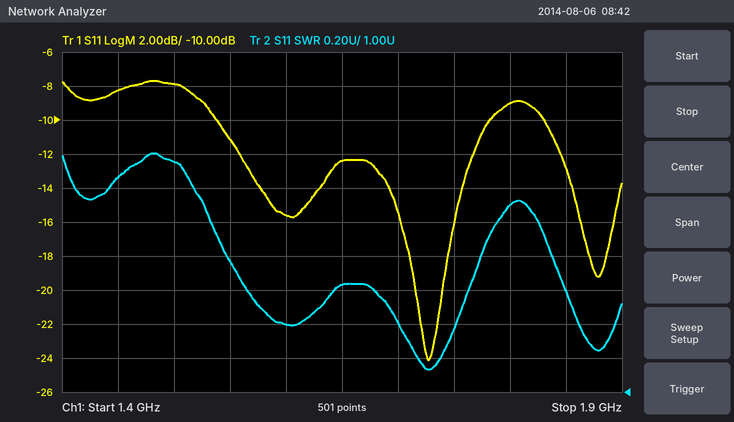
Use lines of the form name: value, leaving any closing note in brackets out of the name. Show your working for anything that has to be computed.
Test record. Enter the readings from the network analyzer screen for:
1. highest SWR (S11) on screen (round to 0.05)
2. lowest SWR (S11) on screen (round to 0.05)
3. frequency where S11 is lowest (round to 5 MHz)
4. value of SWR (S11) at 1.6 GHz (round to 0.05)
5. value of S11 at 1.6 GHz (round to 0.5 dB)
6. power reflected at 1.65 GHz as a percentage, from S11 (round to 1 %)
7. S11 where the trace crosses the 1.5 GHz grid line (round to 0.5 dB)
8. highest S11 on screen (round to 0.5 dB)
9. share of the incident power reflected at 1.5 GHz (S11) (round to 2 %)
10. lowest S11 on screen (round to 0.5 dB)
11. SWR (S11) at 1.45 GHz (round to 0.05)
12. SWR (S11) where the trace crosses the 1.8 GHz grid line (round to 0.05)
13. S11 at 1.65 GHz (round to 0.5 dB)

highest SWR (S11) on screen: 2.40
lowest SWR (S11) on screen: 1.15
frequency where S11 is lowest: 1.725 GHz
value of SWR (S11) at 1.6 GHz: 1.40
value of S11 at 1.6 GHz: -15.5 dB
power reflected at 1.65 GHz as a percentage, from S11: 10^(-12.5/10) ≈ 6 %
S11 where the trace crosses the 1.5 GHz grid line: -8.0 dB
highest S11 on screen: -7.5 dB
share of the incident power reflected at 1.5 GHz (S11): 10^(-8/10) ≈ 16 %
lowest S11 on screen: -24.0 dB
SWR (S11) at 1.45 GHz: 2.25
SWR (S11) where the trace crosses the 1.8 GHz grid line: 2.10
S11 at 1.65 GHz: -12.5 dB
